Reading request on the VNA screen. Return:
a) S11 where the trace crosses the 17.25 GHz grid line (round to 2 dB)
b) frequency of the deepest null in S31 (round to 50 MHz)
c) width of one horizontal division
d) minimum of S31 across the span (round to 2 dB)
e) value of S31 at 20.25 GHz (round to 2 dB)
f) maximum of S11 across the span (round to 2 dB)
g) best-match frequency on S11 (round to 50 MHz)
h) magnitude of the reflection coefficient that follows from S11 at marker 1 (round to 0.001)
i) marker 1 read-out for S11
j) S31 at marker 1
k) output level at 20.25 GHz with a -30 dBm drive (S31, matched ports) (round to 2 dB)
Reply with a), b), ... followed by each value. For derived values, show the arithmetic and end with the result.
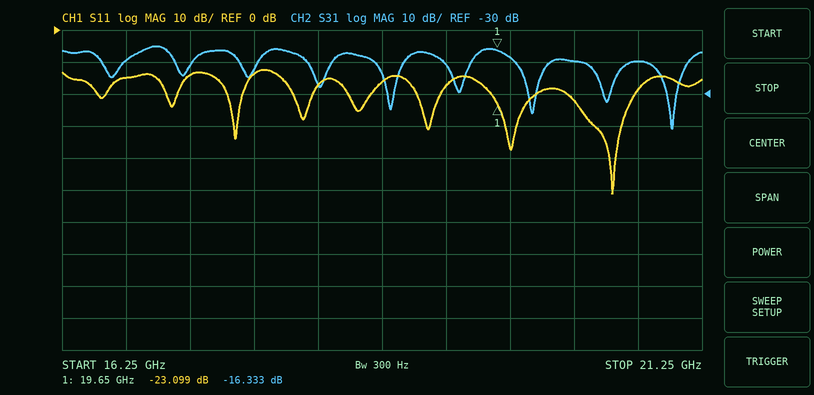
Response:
a) -14 dB
b) 21.00 GHz
c) 500 MHz
d) -40 dB
e) -20 dB
f) -12 dB
g) 20.55 GHz
h) 10^(-23.099/20) ≈ 0.070
i) -23.099 dB
j) -16.333 dB
k) -30 dBm + (-20 dB) = -50 dBm
